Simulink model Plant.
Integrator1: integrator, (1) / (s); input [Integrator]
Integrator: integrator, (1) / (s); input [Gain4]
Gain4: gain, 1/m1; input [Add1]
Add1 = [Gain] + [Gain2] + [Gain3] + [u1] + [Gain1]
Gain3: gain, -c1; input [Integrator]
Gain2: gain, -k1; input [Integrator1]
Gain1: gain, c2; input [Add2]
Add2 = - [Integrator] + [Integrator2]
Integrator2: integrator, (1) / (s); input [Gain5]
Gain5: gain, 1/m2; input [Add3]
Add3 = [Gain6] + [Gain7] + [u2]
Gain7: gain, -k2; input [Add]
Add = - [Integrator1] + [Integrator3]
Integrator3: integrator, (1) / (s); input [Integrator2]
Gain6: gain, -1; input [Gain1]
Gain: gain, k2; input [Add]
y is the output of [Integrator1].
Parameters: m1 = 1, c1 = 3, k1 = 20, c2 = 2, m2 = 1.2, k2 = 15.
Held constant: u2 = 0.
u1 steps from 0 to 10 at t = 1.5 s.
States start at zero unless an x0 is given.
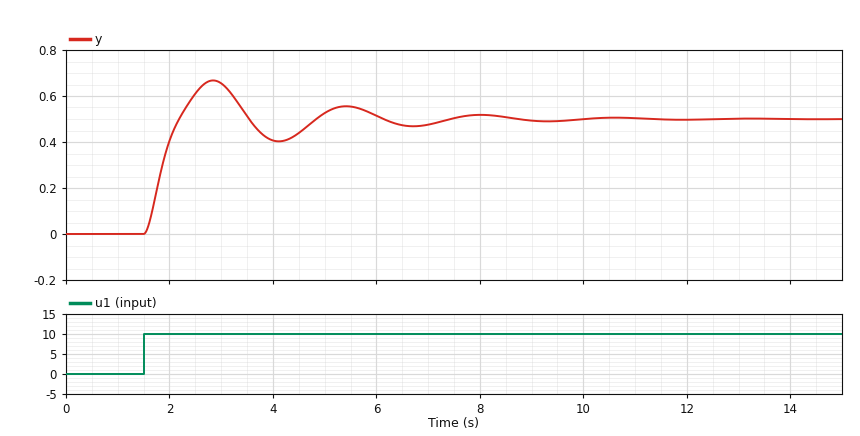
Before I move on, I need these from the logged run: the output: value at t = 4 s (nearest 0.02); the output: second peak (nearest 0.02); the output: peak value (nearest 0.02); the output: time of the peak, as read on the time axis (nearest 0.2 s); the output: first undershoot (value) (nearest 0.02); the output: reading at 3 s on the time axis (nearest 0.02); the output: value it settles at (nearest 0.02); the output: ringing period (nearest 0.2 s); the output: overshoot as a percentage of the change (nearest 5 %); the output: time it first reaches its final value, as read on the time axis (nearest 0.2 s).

0.40
0.56
0.66
2.8 s
0.40
0.66
0.50
2.6 s
35 %
2.2 s
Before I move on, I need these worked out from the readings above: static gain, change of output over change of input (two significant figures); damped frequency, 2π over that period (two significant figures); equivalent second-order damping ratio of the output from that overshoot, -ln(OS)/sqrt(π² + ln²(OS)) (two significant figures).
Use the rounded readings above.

0.050
2.4 rad/s
0.32
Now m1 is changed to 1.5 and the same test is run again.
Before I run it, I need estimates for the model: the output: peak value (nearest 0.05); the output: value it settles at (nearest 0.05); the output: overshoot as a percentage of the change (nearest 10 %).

0.70
0.50
40 %
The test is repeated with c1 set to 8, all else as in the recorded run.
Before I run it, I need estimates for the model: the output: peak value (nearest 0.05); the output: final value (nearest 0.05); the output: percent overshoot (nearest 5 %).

0.55
0.50
15 %
